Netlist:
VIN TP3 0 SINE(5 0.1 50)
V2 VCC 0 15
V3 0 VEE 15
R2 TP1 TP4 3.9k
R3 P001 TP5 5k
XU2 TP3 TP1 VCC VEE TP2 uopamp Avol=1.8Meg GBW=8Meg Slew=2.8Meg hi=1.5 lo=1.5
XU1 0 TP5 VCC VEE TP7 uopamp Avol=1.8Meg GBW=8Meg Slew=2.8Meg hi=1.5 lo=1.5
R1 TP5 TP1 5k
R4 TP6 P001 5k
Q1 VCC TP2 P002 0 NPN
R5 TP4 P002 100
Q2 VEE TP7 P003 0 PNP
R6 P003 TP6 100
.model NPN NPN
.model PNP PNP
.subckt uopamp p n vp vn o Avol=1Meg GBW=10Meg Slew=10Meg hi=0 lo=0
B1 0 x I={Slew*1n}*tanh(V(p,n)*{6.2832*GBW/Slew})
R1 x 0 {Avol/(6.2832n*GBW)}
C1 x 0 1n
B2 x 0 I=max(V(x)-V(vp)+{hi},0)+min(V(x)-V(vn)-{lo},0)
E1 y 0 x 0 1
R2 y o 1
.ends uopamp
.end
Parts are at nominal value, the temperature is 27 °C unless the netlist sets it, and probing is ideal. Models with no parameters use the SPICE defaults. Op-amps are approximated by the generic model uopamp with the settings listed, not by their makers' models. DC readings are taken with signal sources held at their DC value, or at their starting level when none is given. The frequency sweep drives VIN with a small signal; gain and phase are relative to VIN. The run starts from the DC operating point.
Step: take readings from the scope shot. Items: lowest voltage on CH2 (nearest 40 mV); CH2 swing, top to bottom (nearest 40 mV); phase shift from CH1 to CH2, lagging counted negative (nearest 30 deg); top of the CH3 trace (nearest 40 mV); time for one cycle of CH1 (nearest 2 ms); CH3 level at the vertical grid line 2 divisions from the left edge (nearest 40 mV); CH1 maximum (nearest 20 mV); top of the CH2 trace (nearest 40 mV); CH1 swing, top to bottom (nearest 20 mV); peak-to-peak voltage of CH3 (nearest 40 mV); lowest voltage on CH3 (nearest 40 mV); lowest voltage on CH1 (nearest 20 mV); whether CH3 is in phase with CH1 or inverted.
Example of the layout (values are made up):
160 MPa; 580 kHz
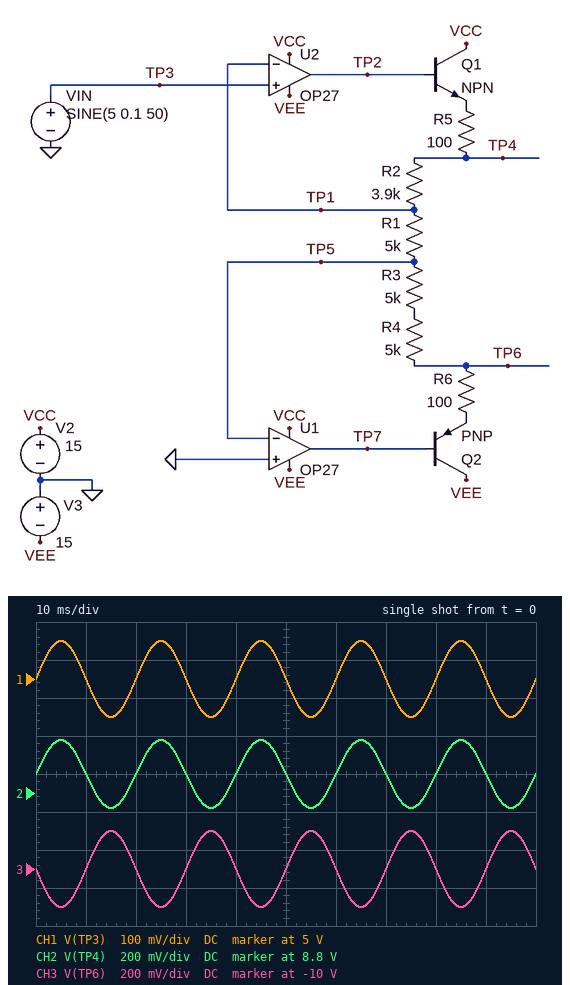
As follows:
8.72 V; 360 mV; 0 deg; -9.80 V; 20 ms; -10.00 V; 5.10 V; 9.08 V; 200 mV; 400 mV; -10.20 V; 4.90 V; inverted
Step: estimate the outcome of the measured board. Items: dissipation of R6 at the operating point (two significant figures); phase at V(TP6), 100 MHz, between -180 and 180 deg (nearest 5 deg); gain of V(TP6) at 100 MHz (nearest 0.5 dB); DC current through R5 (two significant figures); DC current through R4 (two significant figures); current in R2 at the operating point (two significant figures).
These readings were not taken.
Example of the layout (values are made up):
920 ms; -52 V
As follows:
100 µW; -5 deg; -49.5 dB; 1.0 mA; 1.0 mA; 1.0 mA
